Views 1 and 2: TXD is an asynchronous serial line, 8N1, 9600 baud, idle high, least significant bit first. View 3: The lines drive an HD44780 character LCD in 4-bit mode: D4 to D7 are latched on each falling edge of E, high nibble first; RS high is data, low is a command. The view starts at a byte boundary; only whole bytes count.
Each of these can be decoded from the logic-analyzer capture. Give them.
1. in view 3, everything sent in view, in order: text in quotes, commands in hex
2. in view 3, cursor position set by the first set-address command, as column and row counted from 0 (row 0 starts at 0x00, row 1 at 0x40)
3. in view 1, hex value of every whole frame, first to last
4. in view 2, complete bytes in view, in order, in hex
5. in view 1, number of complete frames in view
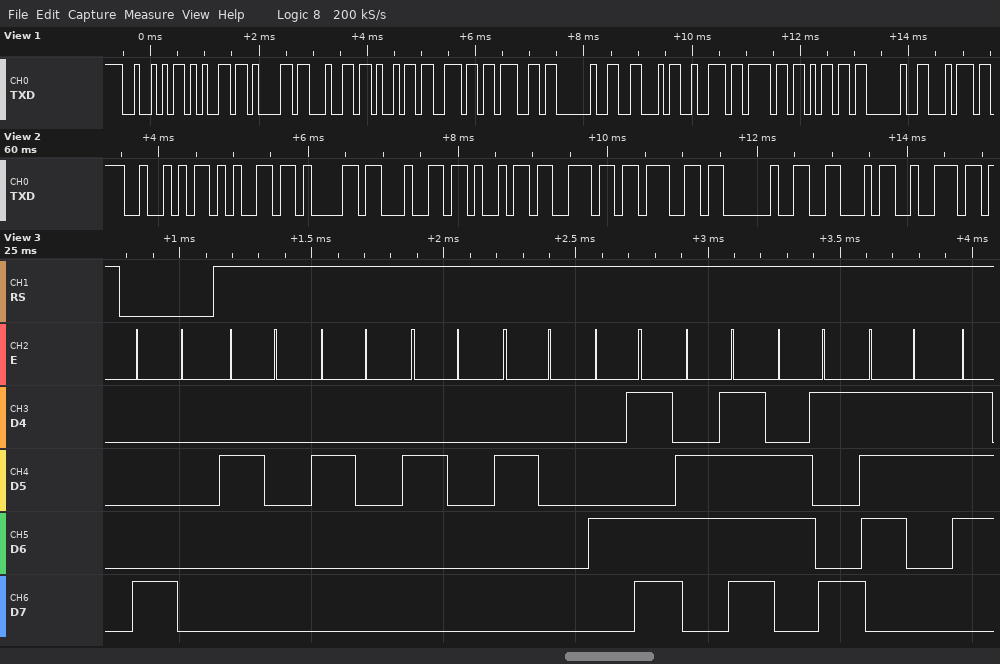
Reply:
0x80 "    Mois"
column 0, row 0
0x52 0x65 0x61 0x64 0x69 0x6E 0x67 0x20 0x46 0x72 0x6F 0x6D 0x20 0x74
52 65 61 64 69 6E 67 20 46 72
14
